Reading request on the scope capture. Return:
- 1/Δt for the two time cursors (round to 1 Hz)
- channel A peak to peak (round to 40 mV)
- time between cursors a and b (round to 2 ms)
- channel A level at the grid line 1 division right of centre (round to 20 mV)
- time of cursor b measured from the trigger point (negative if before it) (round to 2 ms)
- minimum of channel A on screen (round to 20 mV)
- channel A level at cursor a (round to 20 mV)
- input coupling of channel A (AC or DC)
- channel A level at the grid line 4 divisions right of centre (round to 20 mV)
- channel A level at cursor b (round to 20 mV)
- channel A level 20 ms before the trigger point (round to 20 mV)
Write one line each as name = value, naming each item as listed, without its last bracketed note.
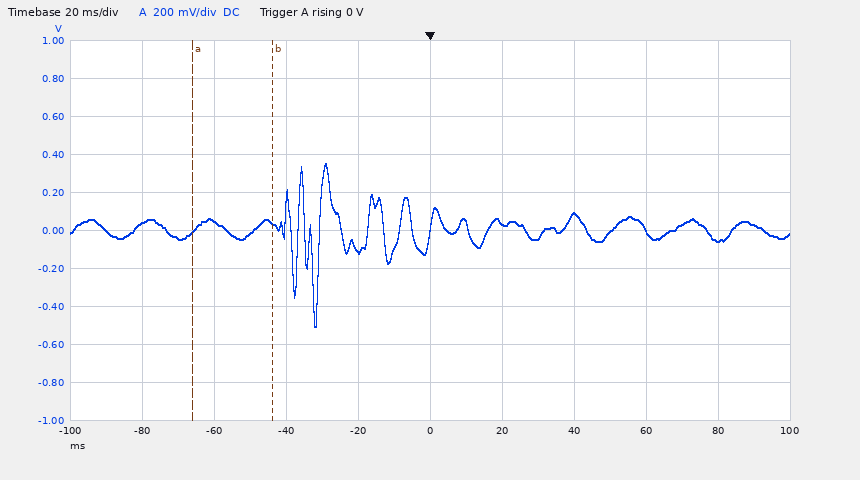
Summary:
1/Δt for the two time cursors = 45 Hz
channel A peak to peak = 840 mV
time between cursors a and b = 22 ms
channel A level at the grid line 1 division right of centre = 40 mV
time of cursor b measured from the trigger point (negative if before it) = -44 ms
minimum of channel A on screen = -500 mV
channel A level at cursor a = 0 mV
input coupling of channel A = DC
channel A level at the grid line 4 divisions right of centre = -60 mV
channel A level at cursor b = 40 mV
channel A level 20 ms before the trigger point = -100 mV
